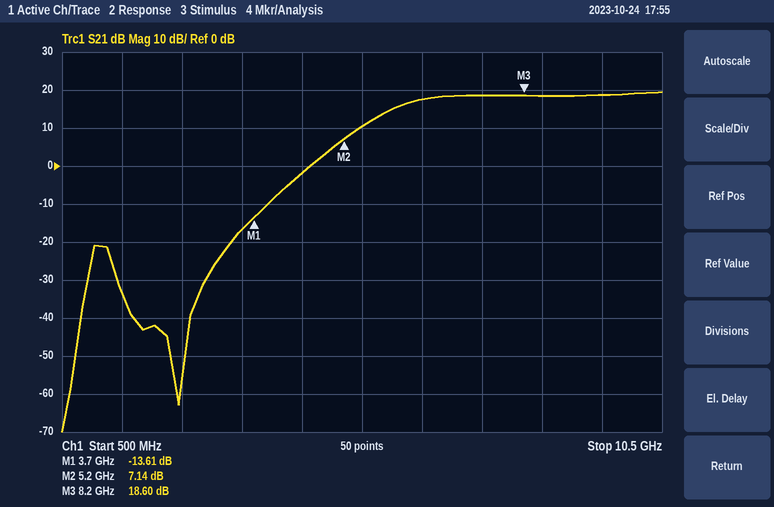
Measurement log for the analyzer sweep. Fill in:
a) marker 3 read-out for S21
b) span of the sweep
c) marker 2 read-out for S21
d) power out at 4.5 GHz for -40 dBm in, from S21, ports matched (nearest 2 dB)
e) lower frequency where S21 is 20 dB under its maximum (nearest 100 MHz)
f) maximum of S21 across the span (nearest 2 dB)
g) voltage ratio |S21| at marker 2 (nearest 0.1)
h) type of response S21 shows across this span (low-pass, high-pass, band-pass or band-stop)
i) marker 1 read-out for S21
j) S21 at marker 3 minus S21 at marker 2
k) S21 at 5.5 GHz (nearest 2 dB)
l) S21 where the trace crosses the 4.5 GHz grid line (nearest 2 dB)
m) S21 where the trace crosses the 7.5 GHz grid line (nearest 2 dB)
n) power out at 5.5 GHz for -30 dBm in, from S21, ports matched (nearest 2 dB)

18.60 dB
10 GHz
7.14 dB
-42 dBm
4.6 GHz
20 dB
2.3
high-pass
-13.61 dB
11.46 dB
10 dB
-2 dB
18 dB
-20 dBm
